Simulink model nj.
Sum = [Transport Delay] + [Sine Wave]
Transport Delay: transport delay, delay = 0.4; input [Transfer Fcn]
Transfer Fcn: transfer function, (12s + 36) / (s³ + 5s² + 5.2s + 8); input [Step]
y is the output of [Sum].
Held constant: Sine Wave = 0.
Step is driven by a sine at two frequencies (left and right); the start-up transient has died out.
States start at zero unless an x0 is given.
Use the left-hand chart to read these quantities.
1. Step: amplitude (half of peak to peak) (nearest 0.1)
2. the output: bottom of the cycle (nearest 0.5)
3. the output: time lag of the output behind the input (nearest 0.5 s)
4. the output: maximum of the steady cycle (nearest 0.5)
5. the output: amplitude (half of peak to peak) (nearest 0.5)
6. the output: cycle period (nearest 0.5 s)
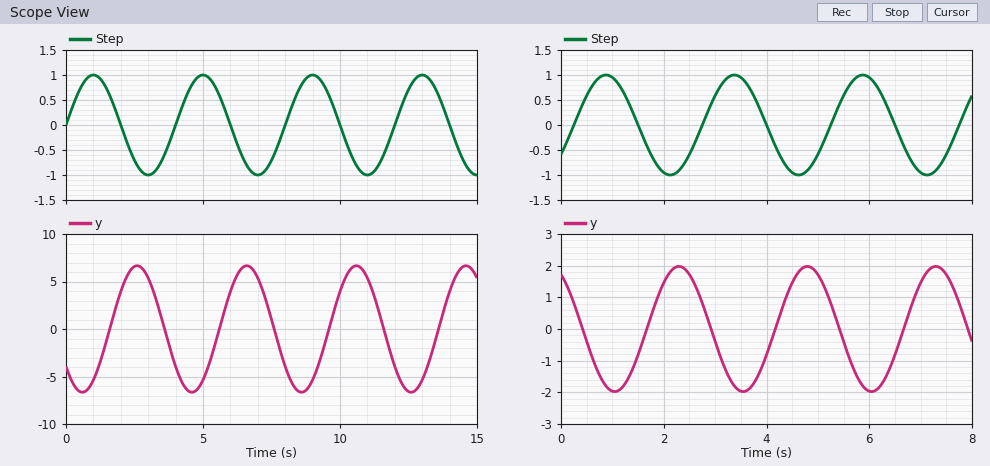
1.0
-6.5
1.5 s
6.5
6.5
4.0 s
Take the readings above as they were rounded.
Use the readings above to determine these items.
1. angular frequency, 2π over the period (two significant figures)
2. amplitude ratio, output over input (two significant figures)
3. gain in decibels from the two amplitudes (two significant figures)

1.6 rad/s
6.5
16 dB
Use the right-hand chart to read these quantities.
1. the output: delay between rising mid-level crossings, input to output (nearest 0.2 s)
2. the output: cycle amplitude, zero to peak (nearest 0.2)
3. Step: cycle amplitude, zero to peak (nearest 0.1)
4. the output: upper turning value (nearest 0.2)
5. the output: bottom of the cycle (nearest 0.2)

1.4 s
2.0
1.0
2.0
-2.0
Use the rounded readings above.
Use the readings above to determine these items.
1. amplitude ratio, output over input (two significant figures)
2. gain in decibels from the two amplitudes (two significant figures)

2.0
6.0 dB
